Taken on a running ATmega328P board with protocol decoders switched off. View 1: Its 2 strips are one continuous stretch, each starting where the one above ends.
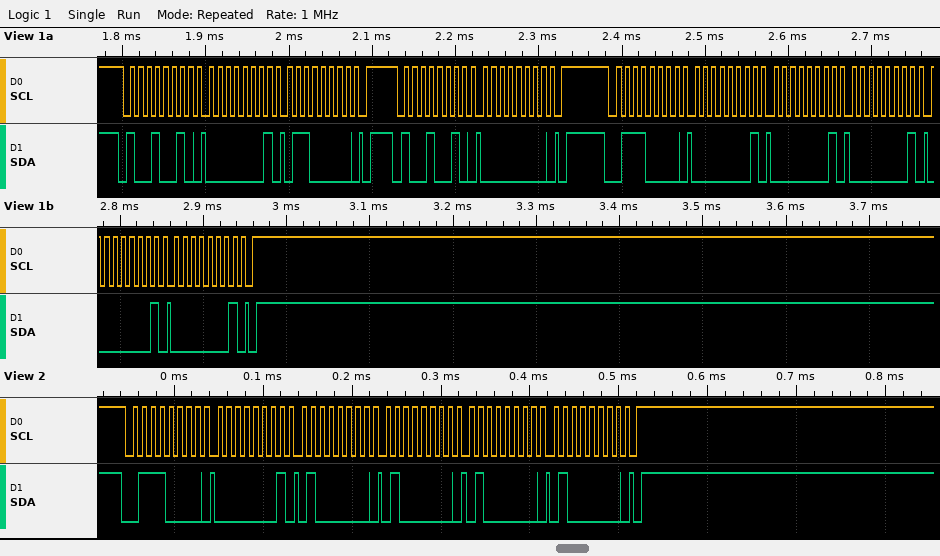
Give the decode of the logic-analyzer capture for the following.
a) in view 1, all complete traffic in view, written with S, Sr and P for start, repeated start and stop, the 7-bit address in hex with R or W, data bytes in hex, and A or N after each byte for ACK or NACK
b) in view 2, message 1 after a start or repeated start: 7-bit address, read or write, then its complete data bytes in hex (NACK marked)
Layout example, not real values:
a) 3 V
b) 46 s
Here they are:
a) S 49W A 01 A 60 A P S 49W A 00 A P S 38W A 01 A 01 A 01 A 01 A 01 A P
b) 0x38 write: 01 40 40 40 40
